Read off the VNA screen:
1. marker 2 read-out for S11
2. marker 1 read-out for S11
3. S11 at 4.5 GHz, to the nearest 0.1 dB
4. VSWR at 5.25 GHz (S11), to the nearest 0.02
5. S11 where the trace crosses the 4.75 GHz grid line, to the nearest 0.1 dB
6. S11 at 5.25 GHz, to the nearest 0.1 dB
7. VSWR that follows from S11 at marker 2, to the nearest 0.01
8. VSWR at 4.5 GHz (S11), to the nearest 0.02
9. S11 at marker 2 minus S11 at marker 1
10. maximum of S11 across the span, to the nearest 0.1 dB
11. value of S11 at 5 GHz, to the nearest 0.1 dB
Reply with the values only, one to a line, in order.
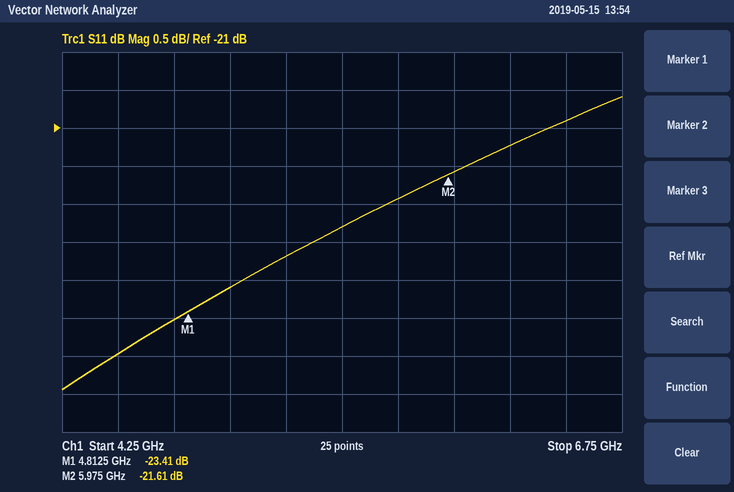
-21.61 dB
-23.41 dB
-24.0 dB
1.16
-23.5 dB
-22.7 dB
1.18
1.14
1.80 dB
-20.6 dB
-23.1 dB
